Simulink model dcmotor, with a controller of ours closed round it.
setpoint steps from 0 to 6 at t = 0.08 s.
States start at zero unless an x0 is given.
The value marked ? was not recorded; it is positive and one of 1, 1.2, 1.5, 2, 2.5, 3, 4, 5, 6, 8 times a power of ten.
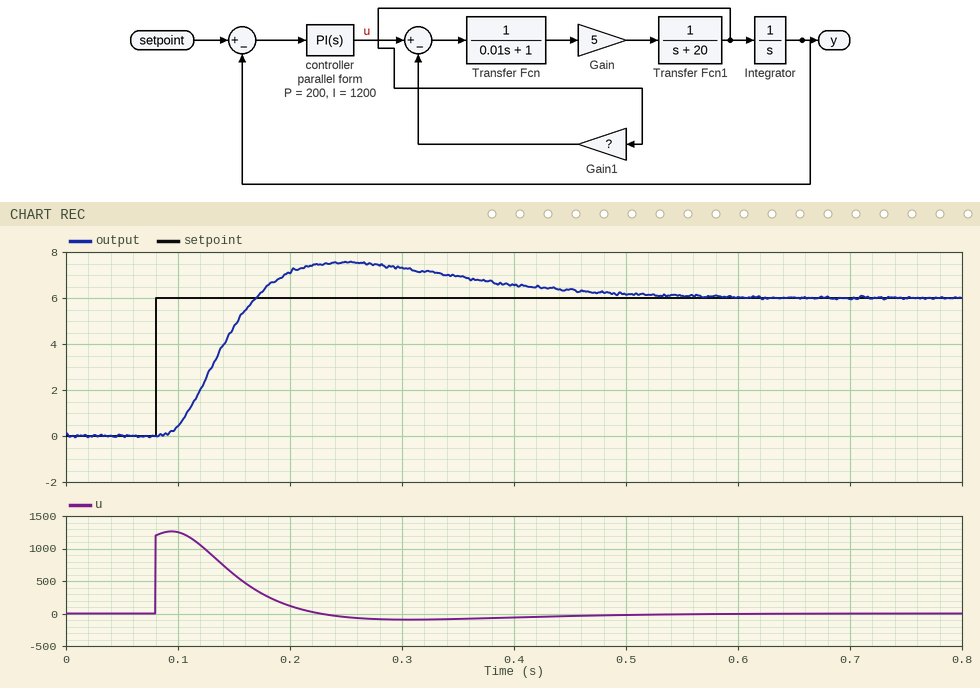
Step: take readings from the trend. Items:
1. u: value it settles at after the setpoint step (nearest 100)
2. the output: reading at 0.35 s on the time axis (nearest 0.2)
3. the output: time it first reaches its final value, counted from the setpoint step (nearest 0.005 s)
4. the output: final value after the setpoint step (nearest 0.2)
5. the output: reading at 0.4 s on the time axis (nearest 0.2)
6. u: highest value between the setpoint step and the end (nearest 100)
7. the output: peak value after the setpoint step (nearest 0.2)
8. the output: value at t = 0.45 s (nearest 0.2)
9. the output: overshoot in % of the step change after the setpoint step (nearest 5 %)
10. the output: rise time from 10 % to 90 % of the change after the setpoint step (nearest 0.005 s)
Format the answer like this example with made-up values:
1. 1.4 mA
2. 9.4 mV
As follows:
1. 0
2. 7.0
3. 0.090 s
4. 6.0
5. 6.6
6. 1300
7. 7.6
8. 6.4
9. 25 %
10. 0.055 s
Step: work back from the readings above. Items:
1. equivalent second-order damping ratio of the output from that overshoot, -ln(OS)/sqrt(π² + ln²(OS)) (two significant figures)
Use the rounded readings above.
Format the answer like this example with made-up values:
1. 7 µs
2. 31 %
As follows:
1. 0.40
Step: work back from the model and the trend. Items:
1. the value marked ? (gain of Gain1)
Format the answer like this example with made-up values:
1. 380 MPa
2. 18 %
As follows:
1. 8
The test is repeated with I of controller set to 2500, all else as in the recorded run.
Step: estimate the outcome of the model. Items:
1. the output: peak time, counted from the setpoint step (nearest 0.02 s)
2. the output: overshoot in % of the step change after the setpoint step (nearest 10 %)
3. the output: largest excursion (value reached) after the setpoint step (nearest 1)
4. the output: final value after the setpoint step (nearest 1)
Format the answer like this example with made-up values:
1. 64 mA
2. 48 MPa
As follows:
1. 0.14 s
2. 50 %
3. 9
4. 6
